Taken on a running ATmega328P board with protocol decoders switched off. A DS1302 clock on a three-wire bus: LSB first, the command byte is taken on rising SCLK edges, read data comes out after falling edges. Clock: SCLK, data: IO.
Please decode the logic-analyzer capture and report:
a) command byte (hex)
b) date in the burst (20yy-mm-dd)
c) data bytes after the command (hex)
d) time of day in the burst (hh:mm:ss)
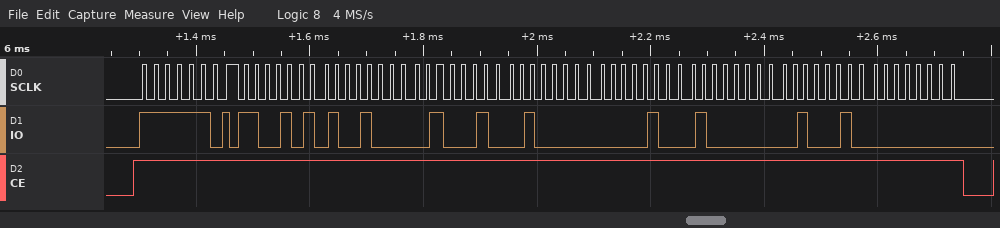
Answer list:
0xBF
2022-10-02
53 09 22 02 10 01 22 00
22:09:53
